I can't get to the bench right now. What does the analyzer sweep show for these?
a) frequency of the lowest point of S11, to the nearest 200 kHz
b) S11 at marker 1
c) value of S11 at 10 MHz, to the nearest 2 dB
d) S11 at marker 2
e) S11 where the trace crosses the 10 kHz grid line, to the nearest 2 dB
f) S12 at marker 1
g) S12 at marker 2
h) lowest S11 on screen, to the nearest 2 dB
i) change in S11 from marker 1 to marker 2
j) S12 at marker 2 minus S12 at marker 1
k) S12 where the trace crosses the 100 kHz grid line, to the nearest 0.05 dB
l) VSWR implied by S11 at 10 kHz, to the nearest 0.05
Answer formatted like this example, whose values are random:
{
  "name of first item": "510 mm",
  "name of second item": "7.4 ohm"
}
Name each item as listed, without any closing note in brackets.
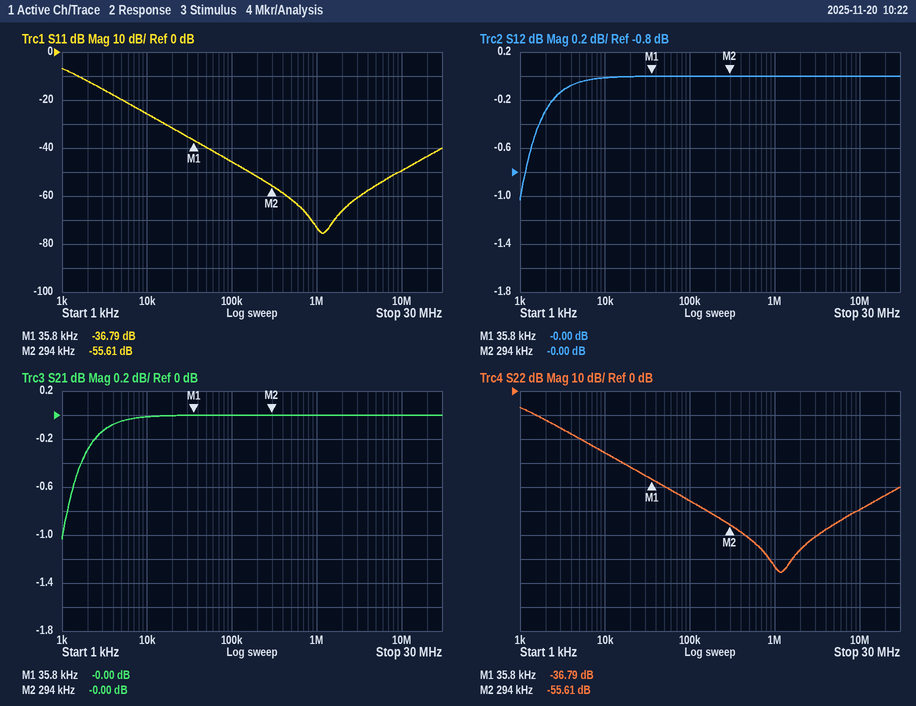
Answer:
{
  "frequency of the lowest point of S11, to the nearest 200 kHz": "1.2 MHz",
  "S11 at marker 1": "-36.79 dB",
  "value of S11 at 10 MHz, to the nearest 2 dB": "-50 dB",
  "S11 at marker 2": "-55.61 dB",
  "S11 where the trace crosses the 10 kHz grid line, to the nearest 2 dB": "-26 dB",
  "S12 at marker 1": "-0.00 dB",
  "S12 at marker 2": "-0.00 dB",
  "lowest S11 on screen, to the nearest 2 dB": "-76 dB",
  "change in S11 from marker 1 to marker 2": "-18.82 dB",
  "S12 at marker 2 minus S12 at marker 1": "0.00 dB",
  "S12 where the trace crosses the 100 kHz grid line, to the nearest 0.05 dB": "0.00 dB",
  "VSWR implied by S11 at 10 kHz, to the nearest 0.05": "1.10"
}
